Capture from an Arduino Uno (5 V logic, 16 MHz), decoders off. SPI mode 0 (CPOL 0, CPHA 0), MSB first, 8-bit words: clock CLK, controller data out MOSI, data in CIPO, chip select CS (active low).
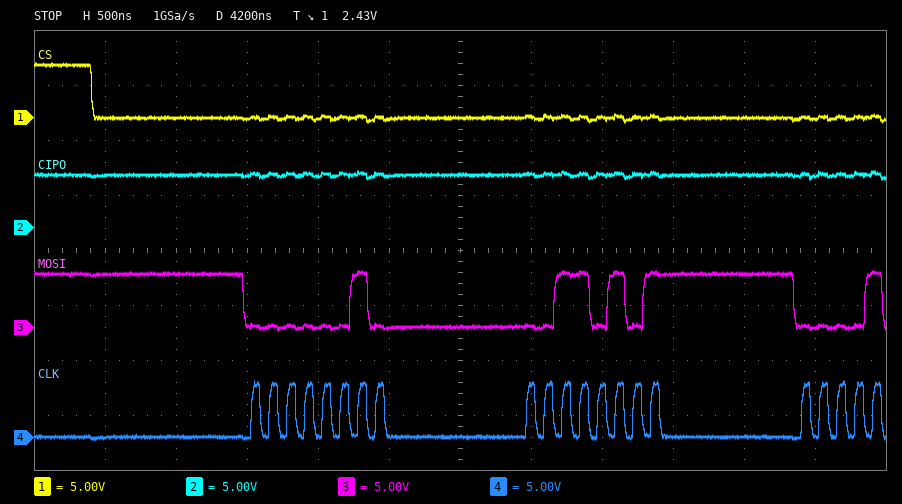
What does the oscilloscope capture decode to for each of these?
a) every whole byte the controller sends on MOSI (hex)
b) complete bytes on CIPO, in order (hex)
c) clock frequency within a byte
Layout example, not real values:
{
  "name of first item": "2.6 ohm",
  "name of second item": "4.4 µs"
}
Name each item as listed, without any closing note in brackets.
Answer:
{
  "every whole byte the controller sends on MOSI": "02 35",
  "complete bytes on CIPO, in order": "FF FF",
  "clock frequency within a byte": "8 MHz"
}
